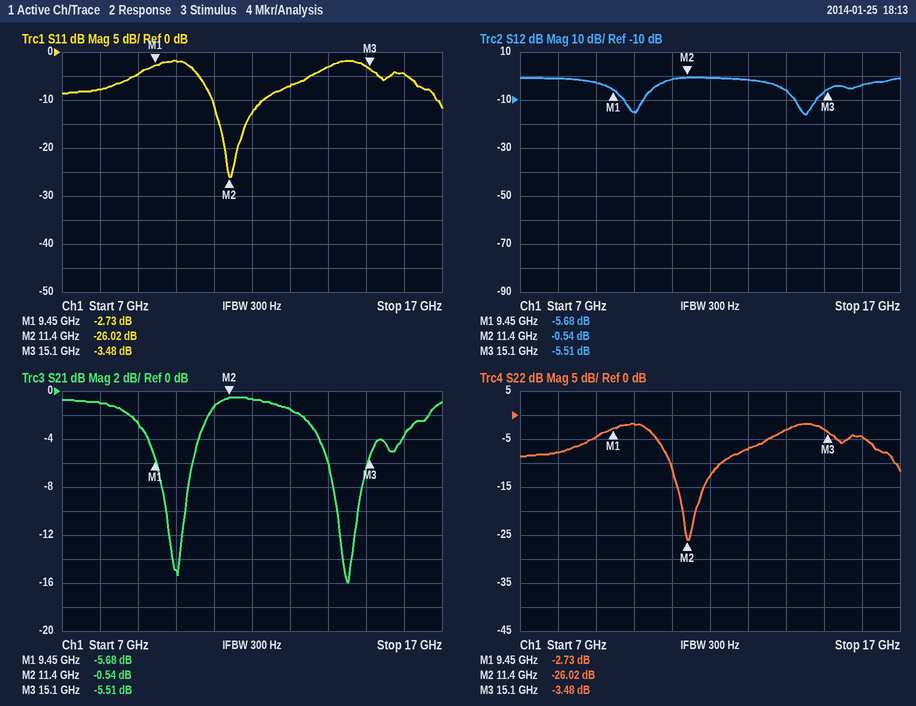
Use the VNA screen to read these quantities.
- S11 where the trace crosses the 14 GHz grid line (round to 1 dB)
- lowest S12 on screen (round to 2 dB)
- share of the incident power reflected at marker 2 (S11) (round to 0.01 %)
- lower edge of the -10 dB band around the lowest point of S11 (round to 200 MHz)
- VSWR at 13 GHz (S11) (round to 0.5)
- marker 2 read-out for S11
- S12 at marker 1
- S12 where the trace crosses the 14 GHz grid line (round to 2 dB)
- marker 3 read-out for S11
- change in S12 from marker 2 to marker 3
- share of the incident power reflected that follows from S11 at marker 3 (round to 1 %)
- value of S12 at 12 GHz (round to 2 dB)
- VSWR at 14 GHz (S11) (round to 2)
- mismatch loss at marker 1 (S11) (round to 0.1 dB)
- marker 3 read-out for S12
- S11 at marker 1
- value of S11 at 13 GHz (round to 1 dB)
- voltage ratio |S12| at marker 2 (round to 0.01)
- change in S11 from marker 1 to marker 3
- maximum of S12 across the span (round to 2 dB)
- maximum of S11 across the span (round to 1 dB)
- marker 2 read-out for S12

-3 dB
-16 dB
0.25 %
11.0 GHz
2.5
-26.02 dB
-5.68 dB
-6 dB
-3.48 dB
-4.97 dB
45 %
0 dB
6
3.3 dB
-5.51 dB
-2.73 dB
-7 dB
0.94
-0.75 dB
0 dB
-2 dB
-0.54 dB
